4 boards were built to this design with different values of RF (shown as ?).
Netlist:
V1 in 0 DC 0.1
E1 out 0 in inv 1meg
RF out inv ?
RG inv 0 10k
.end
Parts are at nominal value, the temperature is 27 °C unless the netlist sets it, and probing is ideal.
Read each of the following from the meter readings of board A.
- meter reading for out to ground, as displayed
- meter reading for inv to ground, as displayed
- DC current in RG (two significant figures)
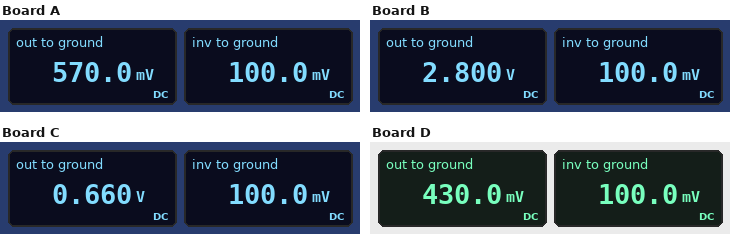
570.0 mV
100.0 mV
10 µA
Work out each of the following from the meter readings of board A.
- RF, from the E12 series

47 kΩ
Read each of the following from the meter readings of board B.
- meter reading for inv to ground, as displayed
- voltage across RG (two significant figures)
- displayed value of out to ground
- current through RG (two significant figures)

100.0 mV
100 mV
2.800 V
10 µA
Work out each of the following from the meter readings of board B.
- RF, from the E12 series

270 kΩ
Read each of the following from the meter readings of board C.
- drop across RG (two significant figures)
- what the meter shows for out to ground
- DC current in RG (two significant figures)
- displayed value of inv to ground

100 mV
0.660 V
10 µA
100.0 mV
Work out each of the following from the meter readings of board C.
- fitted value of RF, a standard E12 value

56 kΩ
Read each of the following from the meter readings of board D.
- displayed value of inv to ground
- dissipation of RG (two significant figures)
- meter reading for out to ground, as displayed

100.0 mV
1.0 µW
430.0 mV
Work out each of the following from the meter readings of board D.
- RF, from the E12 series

33 kΩ
